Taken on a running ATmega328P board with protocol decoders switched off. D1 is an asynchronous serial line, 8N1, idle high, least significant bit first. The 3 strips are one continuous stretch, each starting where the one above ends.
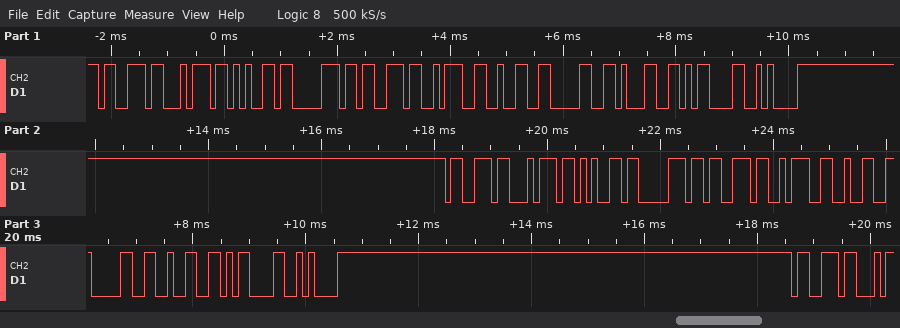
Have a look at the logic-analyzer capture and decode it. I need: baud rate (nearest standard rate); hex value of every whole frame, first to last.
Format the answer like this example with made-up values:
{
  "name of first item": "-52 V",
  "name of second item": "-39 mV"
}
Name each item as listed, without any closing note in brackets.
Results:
{
  "baud rate": "9600 baud",
  "hex value of every whole frame, first to last": "0x73 0x74 0x65 0x70 0x73 0x3A 0x32 0x30 0x31 0x0D 0x0A 0x73 0x74 0x65 0x70 0x73 0x3A 0x32 0x30 0x32 0x0D 0x0A 0x73"
}
